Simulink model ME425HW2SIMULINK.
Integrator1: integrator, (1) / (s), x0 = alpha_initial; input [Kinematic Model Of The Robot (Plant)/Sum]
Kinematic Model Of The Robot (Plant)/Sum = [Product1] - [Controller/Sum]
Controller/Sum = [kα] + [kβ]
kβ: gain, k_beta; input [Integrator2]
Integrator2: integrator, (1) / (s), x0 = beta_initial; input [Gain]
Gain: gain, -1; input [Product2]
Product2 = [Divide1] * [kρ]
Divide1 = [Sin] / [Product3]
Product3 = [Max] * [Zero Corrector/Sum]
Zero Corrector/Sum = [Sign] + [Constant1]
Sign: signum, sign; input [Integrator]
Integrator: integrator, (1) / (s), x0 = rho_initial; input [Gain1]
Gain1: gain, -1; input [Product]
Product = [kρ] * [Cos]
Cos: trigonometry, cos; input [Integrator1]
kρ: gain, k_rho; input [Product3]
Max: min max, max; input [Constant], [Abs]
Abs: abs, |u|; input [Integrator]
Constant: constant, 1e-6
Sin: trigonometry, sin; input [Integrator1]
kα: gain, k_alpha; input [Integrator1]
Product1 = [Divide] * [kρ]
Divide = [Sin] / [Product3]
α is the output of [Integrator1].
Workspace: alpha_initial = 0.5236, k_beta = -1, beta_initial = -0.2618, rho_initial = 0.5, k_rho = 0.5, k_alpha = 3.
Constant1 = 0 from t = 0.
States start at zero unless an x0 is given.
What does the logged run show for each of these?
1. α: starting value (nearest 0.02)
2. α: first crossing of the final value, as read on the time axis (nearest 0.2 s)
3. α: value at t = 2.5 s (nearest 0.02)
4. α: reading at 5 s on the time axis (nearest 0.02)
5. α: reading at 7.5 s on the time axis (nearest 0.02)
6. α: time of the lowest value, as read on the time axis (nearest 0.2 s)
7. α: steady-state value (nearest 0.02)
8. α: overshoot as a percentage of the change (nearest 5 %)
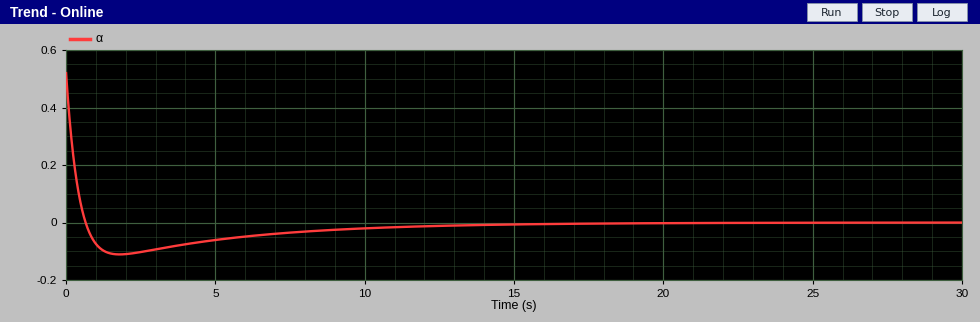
0.52
0.6 s
-0.10
-0.06
-0.04
1.8 s
0.00
20 %
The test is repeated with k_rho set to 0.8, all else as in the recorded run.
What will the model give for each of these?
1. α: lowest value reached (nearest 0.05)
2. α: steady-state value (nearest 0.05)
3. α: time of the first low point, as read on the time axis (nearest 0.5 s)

-0.15
0.00
1.5 s
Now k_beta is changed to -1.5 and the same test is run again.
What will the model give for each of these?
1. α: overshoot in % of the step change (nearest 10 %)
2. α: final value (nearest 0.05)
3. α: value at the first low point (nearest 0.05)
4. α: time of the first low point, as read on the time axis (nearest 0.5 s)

30 %
0.00
-0.15
1.5 s
